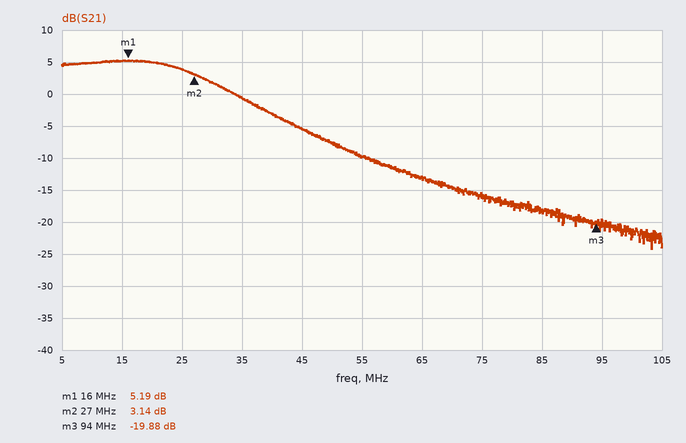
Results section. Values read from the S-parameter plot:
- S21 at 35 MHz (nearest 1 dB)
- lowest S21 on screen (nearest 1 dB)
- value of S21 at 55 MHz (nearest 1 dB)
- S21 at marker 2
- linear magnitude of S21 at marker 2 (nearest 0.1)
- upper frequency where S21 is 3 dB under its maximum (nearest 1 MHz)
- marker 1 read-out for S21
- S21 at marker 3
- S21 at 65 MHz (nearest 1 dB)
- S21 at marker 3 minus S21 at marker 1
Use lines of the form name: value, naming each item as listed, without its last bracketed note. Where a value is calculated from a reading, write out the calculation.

S21 at 35 MHz: -1 dB
lowest S21 on screen: -24 dB
value of S21 at 55 MHz: -10 dB
S21 at marker 2: 3.14 dB
linear magnitude of S21 at marker 2: 10^(3.14/20) ≈ 1.4
upper frequency where S21 is 3 dB under its maximum: 29 MHz
marker 1 read-out for S21: 5.19 dB
S21 at marker 3: -19.88 dB
S21 at 65 MHz: -13 dB
S21 at marker 3 minus S21 at marker 1: -19.88 − (5.19) = -25.07 dB
